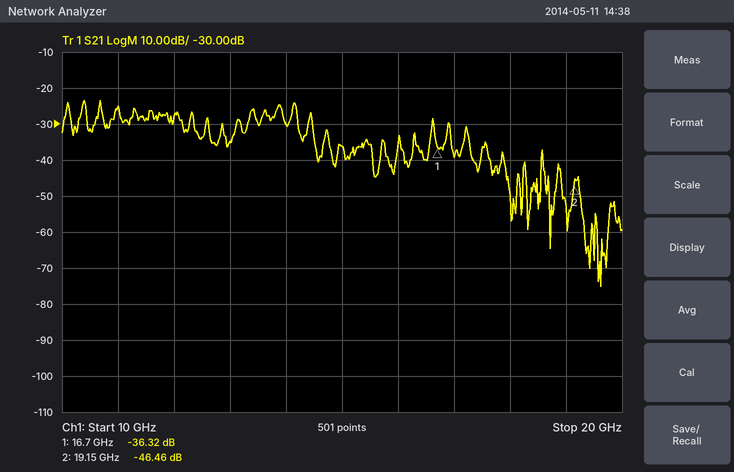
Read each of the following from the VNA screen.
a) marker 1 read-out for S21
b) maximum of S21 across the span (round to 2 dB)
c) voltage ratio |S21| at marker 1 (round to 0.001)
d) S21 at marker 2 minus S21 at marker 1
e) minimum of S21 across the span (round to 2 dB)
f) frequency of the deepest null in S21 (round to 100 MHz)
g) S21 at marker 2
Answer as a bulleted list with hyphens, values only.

- -36.32 dB
- -24 dB
- 0.015
- -10.14 dB
- -76 dB
- 19.6 GHz
- -46.46 dB
